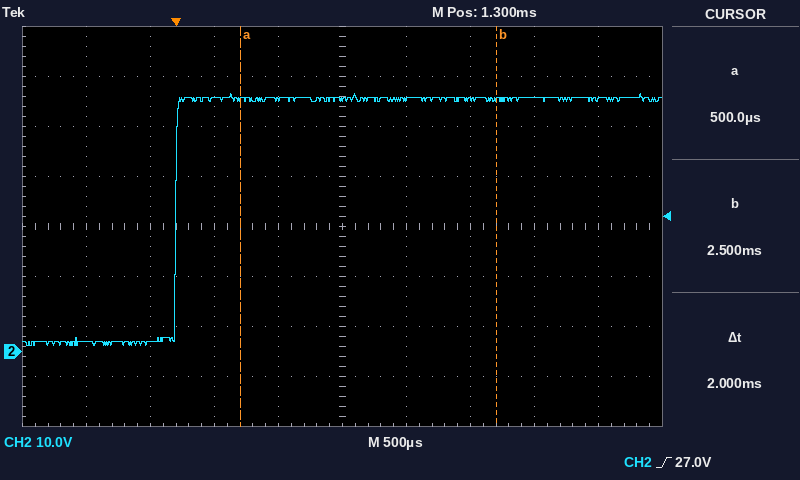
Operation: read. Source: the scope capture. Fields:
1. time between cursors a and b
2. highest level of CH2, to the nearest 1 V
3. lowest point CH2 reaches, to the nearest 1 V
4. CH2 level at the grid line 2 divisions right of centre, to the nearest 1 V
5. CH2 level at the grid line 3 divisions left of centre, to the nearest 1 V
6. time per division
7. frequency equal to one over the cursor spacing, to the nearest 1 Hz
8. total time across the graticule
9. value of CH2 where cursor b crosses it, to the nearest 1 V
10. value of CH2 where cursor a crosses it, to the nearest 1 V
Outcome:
2 ms
52 V
1 V
50 V
2 V
500 µs
500 Hz
5 ms
50 V
50 V
